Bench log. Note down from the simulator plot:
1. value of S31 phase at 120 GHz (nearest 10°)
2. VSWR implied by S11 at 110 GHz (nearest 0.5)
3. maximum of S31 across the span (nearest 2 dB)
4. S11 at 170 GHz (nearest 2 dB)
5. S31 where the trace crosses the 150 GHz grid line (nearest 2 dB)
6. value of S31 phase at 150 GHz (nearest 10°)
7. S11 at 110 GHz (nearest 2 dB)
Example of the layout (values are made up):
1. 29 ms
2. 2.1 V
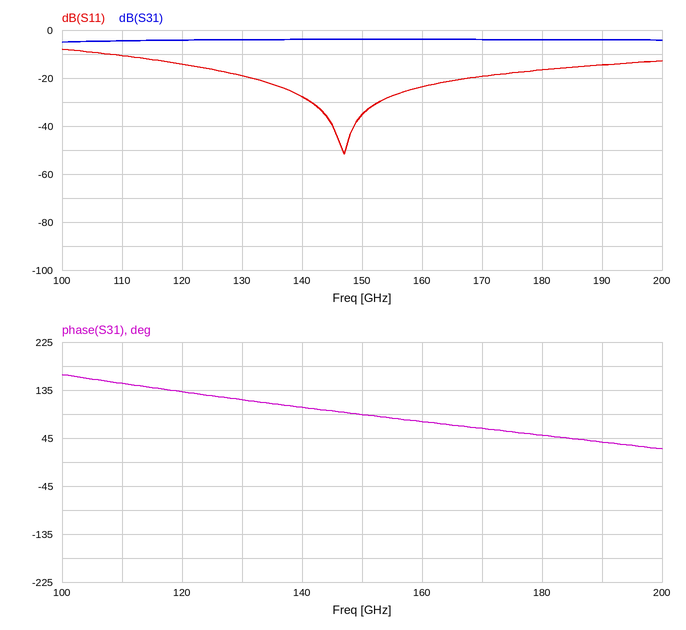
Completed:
1. 130°
2. 2.0
3. -4 dB
4. -20 dB
5. -4 dB
6. 90°
7. -10 dB
